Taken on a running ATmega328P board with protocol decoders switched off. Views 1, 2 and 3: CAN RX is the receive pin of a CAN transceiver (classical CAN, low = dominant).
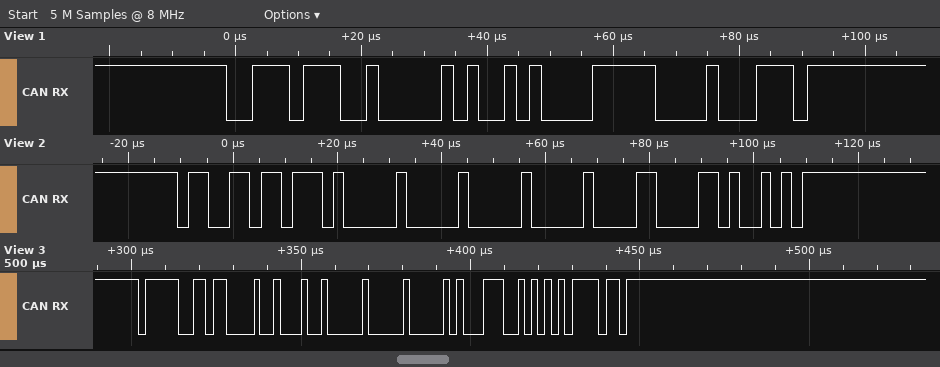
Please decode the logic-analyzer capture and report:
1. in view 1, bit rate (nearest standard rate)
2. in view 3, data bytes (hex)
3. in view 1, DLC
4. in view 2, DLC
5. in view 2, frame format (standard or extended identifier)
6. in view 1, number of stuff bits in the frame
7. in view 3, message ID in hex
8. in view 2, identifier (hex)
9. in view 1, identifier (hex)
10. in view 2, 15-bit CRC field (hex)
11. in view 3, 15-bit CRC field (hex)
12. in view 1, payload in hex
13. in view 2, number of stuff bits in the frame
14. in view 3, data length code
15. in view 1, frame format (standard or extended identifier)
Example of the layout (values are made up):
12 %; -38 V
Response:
500 kbit/s; 89 00 00 8E; 1; 0; extended; 2; 0x7DB; 0x19B50000; 0x3B9; 0x30D2; 0x2ABD; 28; 4; 4; standard
